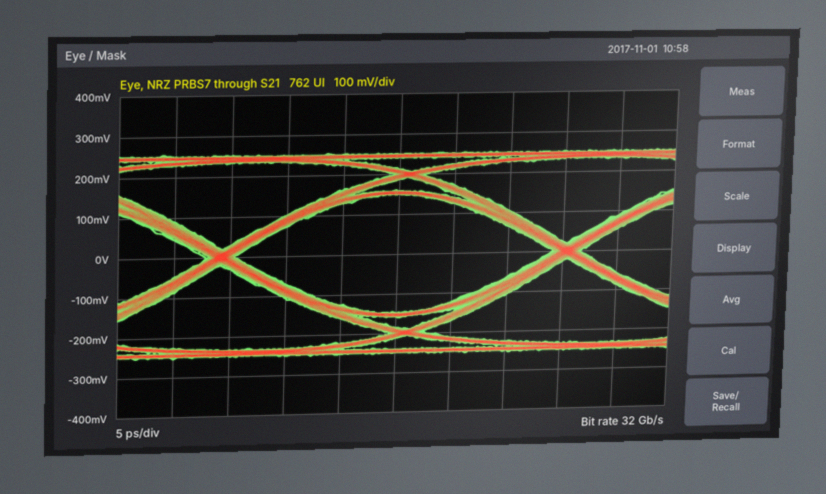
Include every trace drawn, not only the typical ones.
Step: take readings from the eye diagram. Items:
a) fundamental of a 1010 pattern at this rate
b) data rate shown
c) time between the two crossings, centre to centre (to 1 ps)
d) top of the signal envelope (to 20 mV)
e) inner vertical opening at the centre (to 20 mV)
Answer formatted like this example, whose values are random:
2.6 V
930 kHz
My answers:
16 GHz
32 Gb/s
31 ps
260 mV
300 mV
